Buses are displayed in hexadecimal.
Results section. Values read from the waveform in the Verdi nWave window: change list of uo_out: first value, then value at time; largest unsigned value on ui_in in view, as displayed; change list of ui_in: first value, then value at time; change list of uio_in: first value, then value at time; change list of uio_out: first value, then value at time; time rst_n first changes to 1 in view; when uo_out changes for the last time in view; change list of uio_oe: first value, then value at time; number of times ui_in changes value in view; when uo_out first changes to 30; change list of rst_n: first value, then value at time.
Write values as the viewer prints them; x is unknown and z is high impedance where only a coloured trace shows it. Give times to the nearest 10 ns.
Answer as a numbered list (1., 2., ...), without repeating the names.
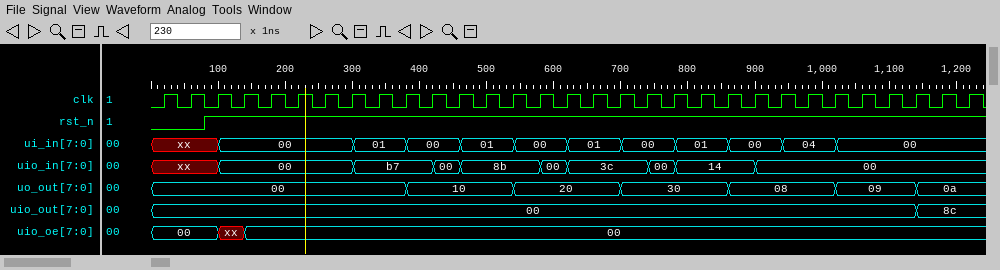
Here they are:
1. 00, 10 at 380 ns, 20 at 540 ns, 30 at 700 ns, 08 at 860 ns, 09 at 1020 ns, 0a at 1140 ns
2. 04
3. xx, 00 at 100 ns, 01 at 300 ns, 00 at 380 ns, 01 at 460 ns, 00 at 540 ns, 01 at 620 ns, 00 at 700 ns, 01 at 780 ns, 00 at 860 ns, 04 at 940 ns, 00 at 1020 ns
4. xx, 00 at 100 ns, b7 at 300 ns, 00 at 420 ns, 8b at 460 ns, 00 at 580 ns, 3c at 620 ns, 00 at 740 ns, 14 at 780 ns, 00 at 900 ns
5. 00, 8c at 1140 ns
6. 80 ns
7. 1140 ns
8. 00, xx at 100 ns, 00 at 140 ns
9. 11
10. 700 ns
11. 0, 1 at 80 ns
